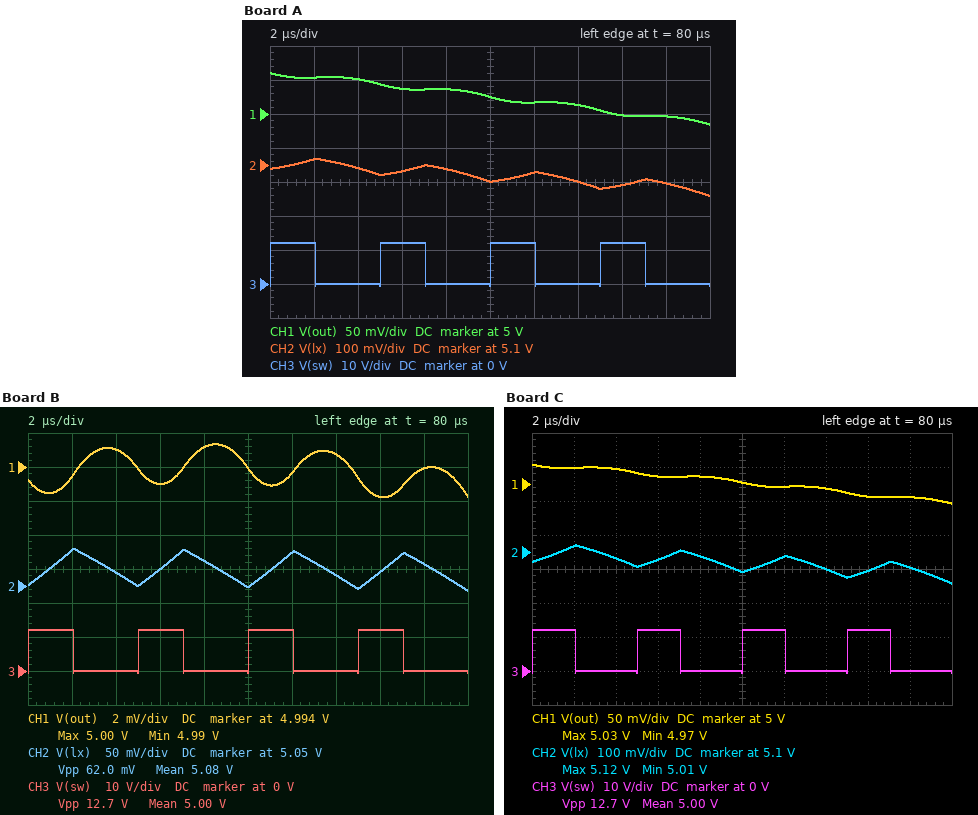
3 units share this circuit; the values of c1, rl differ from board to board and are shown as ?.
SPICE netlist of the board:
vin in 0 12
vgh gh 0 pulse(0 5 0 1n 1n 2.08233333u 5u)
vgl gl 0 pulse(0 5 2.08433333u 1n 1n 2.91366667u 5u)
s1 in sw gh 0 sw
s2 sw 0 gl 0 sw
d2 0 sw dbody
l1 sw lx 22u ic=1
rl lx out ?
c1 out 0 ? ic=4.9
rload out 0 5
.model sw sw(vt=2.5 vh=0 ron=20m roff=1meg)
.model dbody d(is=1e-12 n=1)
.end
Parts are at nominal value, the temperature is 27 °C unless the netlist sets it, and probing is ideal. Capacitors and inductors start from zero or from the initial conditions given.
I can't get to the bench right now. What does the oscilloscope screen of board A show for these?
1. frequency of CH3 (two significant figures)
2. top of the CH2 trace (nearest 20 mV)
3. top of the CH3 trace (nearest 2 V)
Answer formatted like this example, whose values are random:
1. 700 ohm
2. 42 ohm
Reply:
1. 200 kHz
2. 5.12 V
3. 12 V
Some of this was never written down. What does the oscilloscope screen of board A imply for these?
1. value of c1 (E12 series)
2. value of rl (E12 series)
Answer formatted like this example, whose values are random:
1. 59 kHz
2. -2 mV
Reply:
1. 56 µF
2. 0.056 Ω
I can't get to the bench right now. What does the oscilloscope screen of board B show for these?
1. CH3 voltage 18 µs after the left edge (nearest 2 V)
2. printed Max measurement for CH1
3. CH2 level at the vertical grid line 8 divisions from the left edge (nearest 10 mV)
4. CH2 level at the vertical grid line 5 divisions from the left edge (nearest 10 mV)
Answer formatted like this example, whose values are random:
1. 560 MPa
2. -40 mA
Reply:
1. 0 V
2. 5.00 V
3. 5.07 V
4. 5.05 V
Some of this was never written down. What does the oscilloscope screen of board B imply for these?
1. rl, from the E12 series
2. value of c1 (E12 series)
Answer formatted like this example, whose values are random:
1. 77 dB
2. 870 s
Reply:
1. 0.082 Ω
2. 180 µF
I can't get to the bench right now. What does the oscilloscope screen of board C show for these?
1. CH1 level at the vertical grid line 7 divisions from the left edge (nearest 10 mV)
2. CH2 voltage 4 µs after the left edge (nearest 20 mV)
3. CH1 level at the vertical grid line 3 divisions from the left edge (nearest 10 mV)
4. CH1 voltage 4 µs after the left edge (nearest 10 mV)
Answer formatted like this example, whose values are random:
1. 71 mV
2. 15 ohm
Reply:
1. 4.99 V
2. 5.08 V
3. 5.01 V
4. 5.02 V
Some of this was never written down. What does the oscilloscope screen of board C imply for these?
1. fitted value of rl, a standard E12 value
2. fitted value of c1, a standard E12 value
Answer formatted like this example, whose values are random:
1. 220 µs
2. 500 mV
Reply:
1. 0.082 Ω
2. 68 µF
